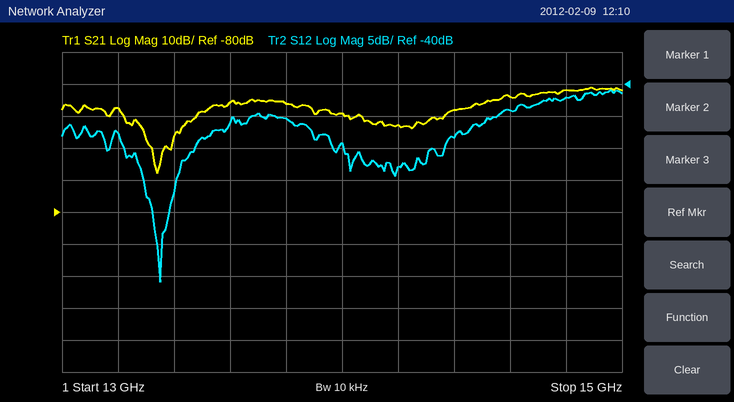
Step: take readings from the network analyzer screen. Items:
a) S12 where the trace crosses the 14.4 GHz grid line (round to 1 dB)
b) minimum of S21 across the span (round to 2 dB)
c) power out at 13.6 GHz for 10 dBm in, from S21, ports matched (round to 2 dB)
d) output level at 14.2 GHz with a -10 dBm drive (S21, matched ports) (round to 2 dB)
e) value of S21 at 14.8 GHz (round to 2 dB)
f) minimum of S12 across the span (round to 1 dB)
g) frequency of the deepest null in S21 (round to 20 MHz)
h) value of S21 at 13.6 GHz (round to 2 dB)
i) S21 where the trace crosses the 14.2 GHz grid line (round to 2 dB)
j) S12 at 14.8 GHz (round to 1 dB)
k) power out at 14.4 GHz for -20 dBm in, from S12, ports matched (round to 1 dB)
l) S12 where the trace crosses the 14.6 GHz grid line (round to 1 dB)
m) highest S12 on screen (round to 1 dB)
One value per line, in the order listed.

-48 dB
-68 dB
-36 dBm
-62 dBm
-42 dB
-71 dB
13.34 GHz
-46 dB
-52 dB
-42 dB
-68 dBm
-44 dB
-41 dB
